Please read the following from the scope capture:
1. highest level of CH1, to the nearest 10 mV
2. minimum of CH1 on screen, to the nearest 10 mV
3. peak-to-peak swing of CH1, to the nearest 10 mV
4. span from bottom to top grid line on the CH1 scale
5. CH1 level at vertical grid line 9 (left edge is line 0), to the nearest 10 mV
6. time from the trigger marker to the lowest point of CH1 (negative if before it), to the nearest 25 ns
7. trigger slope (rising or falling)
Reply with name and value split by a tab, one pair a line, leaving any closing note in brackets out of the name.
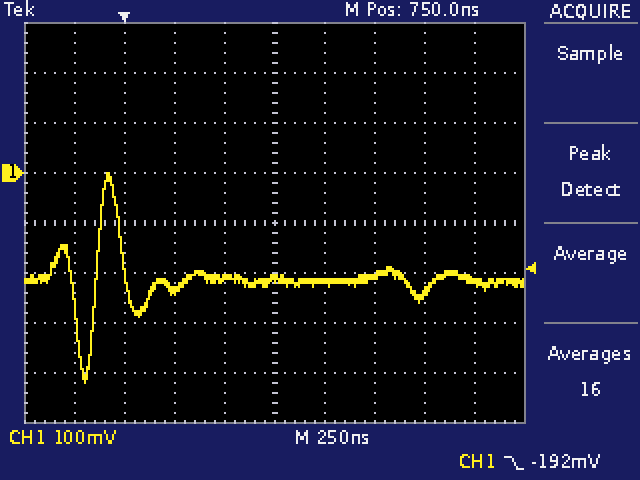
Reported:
highest level of CH1, to the nearest 10 mV	0 mV
minimum of CH1 on screen, to the nearest 10 mV	-420 mV
peak-to-peak swing of CH1, to the nearest 10 mV	420 mV
span from bottom to top grid line on the CH1 scale	800 mV
CH1 level at vertical grid line 9 (left edge is line 0), to the nearest 10 mV	-220 mV
time from the trigger marker to the lowest point of CH1 (negative if before it), to the nearest 25 ns	-200 ns
trigger slope	falling
